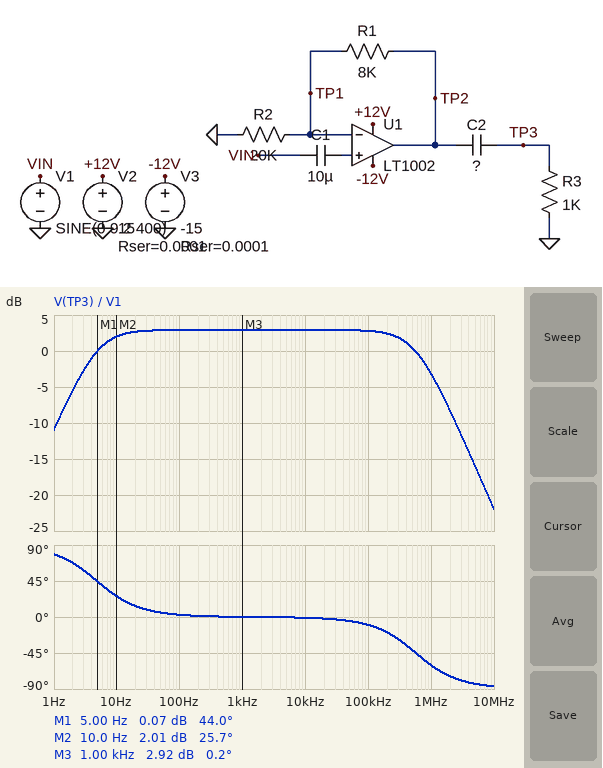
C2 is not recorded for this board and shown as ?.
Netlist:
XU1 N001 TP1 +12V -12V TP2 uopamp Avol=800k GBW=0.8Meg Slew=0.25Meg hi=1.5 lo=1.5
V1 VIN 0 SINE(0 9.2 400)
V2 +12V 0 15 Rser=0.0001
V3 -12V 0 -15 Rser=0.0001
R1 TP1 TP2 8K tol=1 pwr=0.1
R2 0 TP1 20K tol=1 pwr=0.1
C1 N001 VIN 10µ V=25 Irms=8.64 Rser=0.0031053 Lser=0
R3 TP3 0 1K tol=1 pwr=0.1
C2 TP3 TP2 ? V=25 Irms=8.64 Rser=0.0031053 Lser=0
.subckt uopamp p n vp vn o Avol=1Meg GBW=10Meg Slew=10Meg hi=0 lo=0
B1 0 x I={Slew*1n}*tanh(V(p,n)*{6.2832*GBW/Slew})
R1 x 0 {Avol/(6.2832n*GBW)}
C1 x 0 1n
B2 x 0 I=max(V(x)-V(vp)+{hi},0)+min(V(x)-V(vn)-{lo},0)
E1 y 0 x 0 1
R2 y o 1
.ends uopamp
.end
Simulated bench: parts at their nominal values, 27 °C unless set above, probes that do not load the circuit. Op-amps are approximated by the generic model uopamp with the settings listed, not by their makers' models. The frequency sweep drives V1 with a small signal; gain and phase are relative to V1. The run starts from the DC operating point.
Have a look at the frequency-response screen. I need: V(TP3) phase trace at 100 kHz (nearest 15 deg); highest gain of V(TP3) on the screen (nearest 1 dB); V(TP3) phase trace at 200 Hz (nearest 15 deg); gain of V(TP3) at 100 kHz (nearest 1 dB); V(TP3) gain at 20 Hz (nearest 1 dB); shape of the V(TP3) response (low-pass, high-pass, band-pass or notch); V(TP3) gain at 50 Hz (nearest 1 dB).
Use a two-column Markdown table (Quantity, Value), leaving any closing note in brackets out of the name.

| Quantity | Value |
|---|---|
| V(TP3) phase trace at 100 kHz | -15 deg |
| highest gain of V(TP3) on the screen | 3 dB |
| V(TP3) phase trace at 200 Hz | 0 deg |
| gain of V(TP3) at 100 kHz | 3 dB |
| V(TP3) gain at 20 Hz | 3 dB |
| shape of the V(TP3) response | band-pass |
| V(TP3) gain at 50 Hz | 3 dB |
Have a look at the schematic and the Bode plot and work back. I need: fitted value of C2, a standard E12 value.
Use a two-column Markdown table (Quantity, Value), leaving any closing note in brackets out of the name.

| Quantity | Value |
|---|---|
| fitted value of C2, a standard E12 value | 33 µF |
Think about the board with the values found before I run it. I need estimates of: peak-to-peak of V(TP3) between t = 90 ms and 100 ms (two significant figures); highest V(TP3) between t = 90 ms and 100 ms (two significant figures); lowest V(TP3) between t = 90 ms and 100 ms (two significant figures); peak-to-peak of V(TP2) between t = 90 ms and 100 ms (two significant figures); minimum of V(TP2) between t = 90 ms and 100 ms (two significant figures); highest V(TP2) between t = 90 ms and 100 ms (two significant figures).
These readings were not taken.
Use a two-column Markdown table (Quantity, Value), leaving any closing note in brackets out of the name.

| Quantity | Value |
|---|---|
| peak-to-peak of V(TP3) between t = 90 ms and 100 ms | 26 V |
| highest V(TP3) between t = 90 ms and 100 ms | 13 V |
| lowest V(TP3) between t = 90 ms and 100 ms | -13 V |
| peak-to-peak of V(TP2) between t = 90 ms and 100 ms | 26 V |
| minimum of V(TP2) between t = 90 ms and 100 ms | -13 V |
| highest V(TP2) between t = 90 ms and 100 ms | 13 V |
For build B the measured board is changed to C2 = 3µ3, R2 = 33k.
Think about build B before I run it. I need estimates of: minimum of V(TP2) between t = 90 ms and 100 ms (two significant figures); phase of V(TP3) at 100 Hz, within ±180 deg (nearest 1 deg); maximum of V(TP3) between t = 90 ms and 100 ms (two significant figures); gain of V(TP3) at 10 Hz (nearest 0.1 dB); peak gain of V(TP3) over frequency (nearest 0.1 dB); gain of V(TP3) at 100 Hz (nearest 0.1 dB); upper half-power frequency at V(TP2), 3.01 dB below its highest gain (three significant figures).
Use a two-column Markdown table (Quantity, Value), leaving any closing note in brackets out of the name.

| Quantity | Value |
|---|---|
| minimum of V(TP2) between t = 90 ms and 100 ms | -11 V |
| phase of V(TP3) at 100 Hz, within ±180 deg | 26 deg |
| maximum of V(TP3) between t = 90 ms and 100 ms | 11 V |
| gain of V(TP3) at 10 Hz | -12.0 dB |
| peak gain of V(TP3) over frequency | 1.9 dB |
| gain of V(TP3) at 100 Hz | 1.0 dB |
| upper half-power frequency at V(TP2), 3.01 dB below its highest gain | 643 kHz |
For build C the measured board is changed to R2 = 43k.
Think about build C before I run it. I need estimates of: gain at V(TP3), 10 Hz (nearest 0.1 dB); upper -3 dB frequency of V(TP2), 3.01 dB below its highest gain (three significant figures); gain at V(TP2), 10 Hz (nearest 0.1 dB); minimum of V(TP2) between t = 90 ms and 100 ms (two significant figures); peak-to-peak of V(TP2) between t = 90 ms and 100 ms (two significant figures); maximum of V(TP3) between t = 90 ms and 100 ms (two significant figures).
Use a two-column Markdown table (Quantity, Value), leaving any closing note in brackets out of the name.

| Quantity | Value |
|---|---|
| gain at V(TP3), 10 Hz | 0.6 dB |
| upper -3 dB frequency of V(TP2), 3.01 dB below its highest gain | 674 kHz |
| gain at V(TP2), 10 Hz | 1.5 dB |
| minimum of V(TP2) between t = 90 ms and 100 ms | -11 V |
| peak-to-peak of V(TP2) between t = 90 ms and 100 ms | 22 V |
| maximum of V(TP3) between t = 90 ms and 100 ms | 11 V |
